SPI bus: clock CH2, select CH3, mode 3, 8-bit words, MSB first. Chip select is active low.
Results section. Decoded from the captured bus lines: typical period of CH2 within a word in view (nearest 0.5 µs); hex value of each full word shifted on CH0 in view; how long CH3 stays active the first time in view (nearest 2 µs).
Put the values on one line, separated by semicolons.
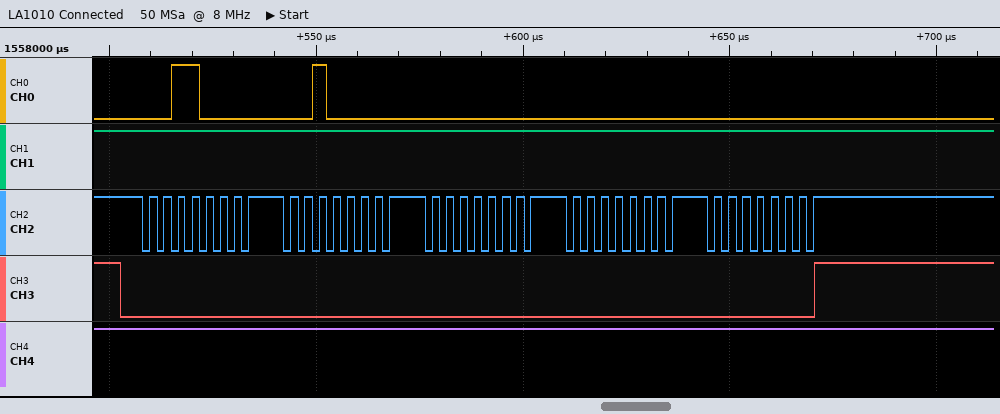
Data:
3.5 µs; 30, 20, 00, 00, 00; 168 µs
